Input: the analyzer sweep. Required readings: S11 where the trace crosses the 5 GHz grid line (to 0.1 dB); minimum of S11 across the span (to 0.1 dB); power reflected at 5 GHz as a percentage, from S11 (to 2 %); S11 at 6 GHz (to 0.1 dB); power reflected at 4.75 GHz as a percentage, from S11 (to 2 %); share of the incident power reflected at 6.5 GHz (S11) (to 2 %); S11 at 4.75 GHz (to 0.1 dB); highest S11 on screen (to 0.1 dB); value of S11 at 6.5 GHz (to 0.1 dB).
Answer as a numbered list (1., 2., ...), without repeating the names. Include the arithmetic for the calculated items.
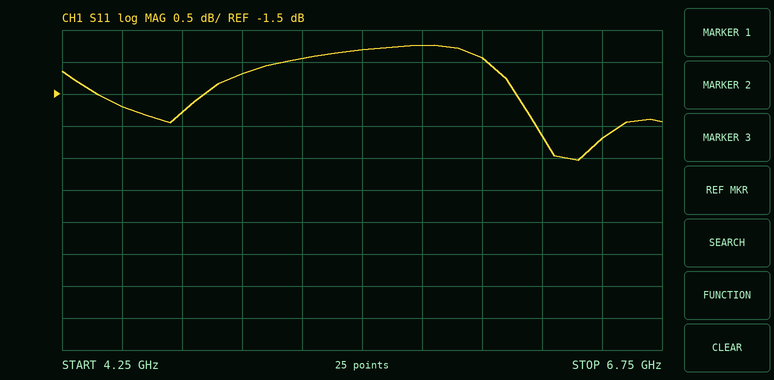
1. -1.2 dB
2. -2.5 dB
3. 10^(-1.2/10) ≈ 76 %
4. -0.9 dB
5. 10^(-1.8/10) ≈ 66 %
6. 10^(-2.2/10) ≈ 60 %
7. -1.8 dB
8. -0.7 dB
9. -2.2 dB
